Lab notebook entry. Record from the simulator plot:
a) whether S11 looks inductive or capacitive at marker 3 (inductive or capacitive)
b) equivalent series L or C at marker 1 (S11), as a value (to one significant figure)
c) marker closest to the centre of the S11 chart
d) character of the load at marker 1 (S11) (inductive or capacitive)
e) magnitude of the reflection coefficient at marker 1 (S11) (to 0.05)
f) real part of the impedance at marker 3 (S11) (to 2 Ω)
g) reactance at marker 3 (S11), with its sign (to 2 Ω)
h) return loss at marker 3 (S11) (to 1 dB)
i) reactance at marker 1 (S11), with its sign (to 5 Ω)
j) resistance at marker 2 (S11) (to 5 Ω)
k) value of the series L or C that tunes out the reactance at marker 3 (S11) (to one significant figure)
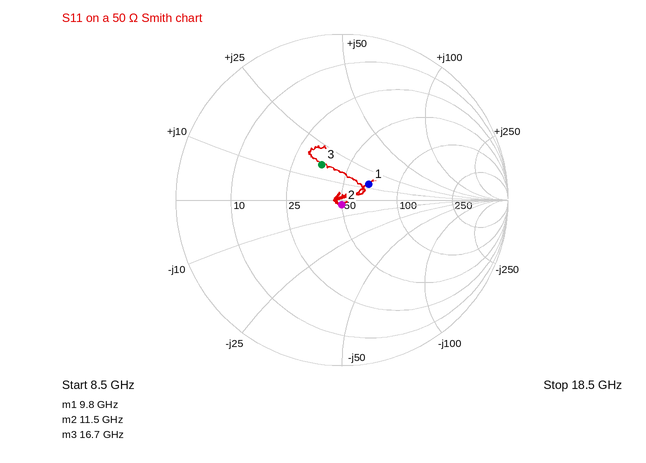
inductive
200 pH
marker 2
inductive
0.20
36 Ω
+16 Ω
12 dB
+15 Ω
50 Ω
600 fF
